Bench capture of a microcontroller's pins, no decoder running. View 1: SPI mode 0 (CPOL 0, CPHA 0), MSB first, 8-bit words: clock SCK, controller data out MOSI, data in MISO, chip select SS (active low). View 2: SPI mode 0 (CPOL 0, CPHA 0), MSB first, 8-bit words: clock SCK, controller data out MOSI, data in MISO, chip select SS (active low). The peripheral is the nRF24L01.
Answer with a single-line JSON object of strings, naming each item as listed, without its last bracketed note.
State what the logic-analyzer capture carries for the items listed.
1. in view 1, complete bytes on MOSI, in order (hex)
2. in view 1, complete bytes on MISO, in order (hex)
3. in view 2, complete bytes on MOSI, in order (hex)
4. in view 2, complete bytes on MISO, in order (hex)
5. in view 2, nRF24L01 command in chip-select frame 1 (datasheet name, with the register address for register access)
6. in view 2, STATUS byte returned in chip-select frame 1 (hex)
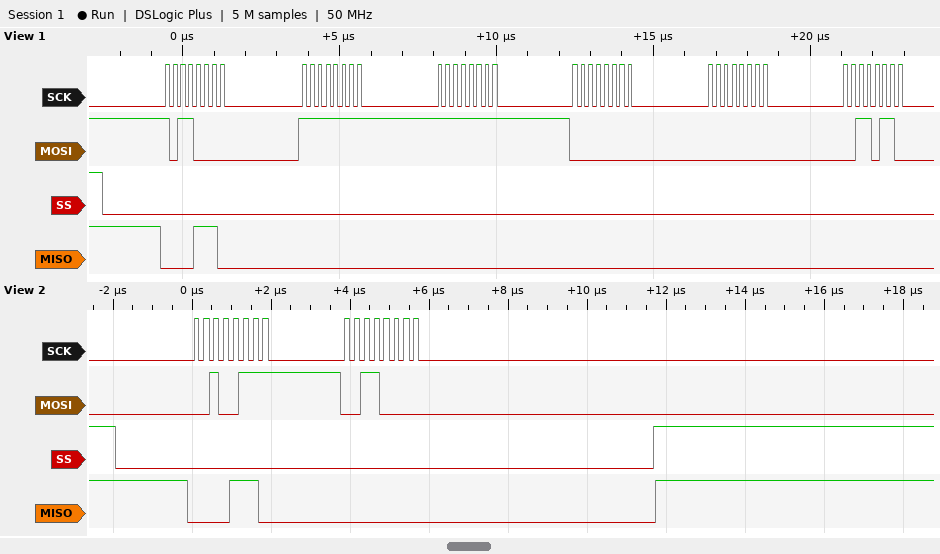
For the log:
{"in view 1, complete bytes on MOSI, in order": "B0 FF FF 00 00 36", "in view 1, complete bytes on MISO, in order": "0E 00 00 00 00 00", "in view 2, complete bytes on MOSI, in order": "27 30", "in view 2, complete bytes on MISO, in order": "0E 00", "in view 2, nRF24L01 command in chip-select frame 1": "W_REGISTER 0x07", "in view 2, STATUS byte returned in chip-select frame 1": "0x0E"}
